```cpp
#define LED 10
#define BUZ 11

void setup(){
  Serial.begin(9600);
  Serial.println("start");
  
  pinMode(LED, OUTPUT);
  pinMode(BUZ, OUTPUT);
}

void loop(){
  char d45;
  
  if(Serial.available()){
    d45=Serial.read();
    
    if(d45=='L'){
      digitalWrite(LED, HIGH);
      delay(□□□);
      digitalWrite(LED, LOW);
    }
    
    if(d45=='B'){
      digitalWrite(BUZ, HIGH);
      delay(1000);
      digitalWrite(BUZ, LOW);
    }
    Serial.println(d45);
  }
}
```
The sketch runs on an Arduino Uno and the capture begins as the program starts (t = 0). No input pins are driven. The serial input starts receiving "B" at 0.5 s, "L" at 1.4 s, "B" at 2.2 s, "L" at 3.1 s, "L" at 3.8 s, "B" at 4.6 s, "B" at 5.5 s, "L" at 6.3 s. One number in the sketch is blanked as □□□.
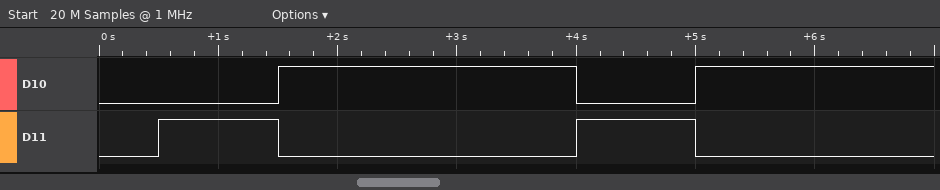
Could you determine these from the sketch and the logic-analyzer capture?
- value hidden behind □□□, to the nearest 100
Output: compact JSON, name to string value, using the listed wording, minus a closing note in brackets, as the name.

{"value hidden behind □□□, to the nearest 100": "2500"}
